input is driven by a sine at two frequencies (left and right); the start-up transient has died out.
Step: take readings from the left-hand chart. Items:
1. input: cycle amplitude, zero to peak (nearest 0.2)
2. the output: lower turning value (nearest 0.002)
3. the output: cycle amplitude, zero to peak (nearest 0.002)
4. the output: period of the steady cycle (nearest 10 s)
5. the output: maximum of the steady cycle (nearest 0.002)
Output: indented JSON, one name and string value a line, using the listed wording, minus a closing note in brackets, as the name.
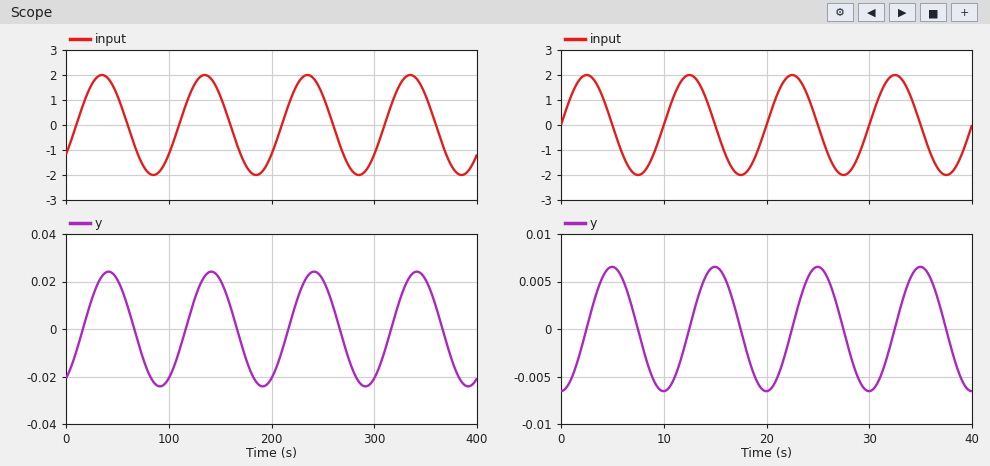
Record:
{
  "input: cycle amplitude, zero to peak": "2.0",
  "the output: lower turning value": "-0.024",
  "the output: cycle amplitude, zero to peak": "0.024",
  "the output: period of the steady cycle": "100 s",
  "the output: maximum of the steady cycle": "0.024"
}
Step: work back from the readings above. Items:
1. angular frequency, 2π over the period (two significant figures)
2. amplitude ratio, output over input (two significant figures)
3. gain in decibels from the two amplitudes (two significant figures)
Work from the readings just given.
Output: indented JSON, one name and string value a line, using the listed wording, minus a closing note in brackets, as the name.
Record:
{
  "angular frequency, 2π over the period": "0.063 rad/s",
  "amplitude ratio, output over input": "0.012",
  "gain in decibels from the two amplitudes": "-38 dB"
}
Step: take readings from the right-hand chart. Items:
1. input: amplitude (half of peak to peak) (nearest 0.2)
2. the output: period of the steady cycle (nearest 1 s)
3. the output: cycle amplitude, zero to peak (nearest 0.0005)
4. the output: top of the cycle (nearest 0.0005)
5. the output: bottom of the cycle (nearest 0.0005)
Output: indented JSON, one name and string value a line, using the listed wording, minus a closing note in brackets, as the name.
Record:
{
  "input: amplitude (half of peak to peak)": "2.0",
  "the output: period of the steady cycle": "10 s",
  "the output: cycle amplitude, zero to peak": "0.0065",
  "the output: top of the cycle": "0.0065",
  "the output: bottom of the cycle": "-0.0065"
}
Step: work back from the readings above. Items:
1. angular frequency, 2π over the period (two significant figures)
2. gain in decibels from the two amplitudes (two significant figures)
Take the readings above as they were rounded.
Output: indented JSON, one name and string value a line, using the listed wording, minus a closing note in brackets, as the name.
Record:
{
  "angular frequency, 2π over the period": "0.63 rad/s",
  "gain in decibels from the two amplitudes": "-50 dB"
}
